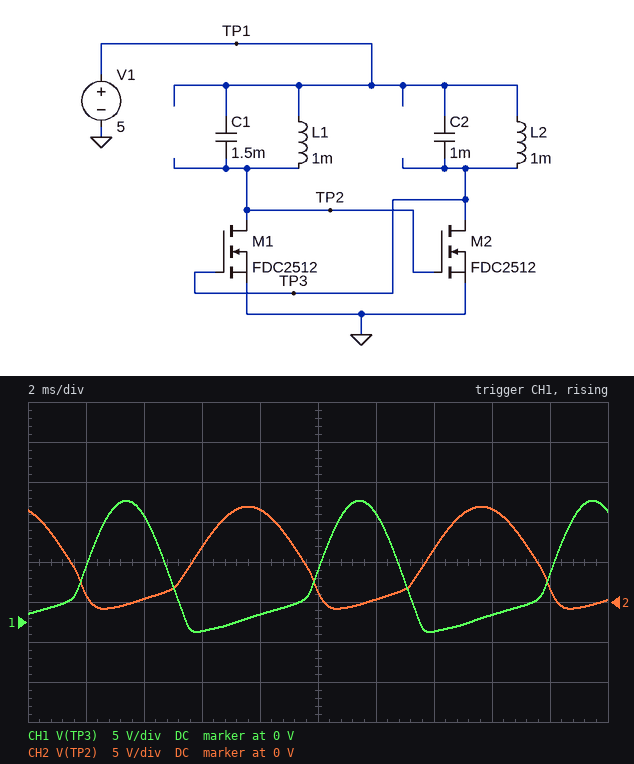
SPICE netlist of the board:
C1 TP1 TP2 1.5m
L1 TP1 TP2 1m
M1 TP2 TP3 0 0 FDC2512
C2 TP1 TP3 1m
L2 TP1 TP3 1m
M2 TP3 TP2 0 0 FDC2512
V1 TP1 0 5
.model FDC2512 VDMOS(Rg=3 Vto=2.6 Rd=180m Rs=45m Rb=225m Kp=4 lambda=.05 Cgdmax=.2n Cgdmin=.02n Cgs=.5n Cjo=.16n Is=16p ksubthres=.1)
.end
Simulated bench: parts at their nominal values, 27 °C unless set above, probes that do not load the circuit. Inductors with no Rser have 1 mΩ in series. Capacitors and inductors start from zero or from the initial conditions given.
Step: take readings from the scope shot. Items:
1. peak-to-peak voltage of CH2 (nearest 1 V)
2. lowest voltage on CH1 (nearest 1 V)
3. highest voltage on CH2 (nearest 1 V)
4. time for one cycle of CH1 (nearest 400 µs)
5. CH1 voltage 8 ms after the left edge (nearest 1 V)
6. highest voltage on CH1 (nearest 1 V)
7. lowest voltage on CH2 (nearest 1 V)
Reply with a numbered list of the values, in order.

1. 13 V
2. -1 V
3. 12 V
4. 8.0 ms
5. 1 V
6. 15 V
7. -1 V
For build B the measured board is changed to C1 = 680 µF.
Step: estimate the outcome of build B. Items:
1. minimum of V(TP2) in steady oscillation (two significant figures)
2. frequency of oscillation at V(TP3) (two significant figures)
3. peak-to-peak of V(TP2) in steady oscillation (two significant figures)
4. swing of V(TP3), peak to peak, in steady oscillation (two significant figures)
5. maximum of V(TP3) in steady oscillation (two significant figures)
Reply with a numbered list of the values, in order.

1. -1.2 V
2. 150 Hz
3. 17 V
4. 13 V
5. 12 V
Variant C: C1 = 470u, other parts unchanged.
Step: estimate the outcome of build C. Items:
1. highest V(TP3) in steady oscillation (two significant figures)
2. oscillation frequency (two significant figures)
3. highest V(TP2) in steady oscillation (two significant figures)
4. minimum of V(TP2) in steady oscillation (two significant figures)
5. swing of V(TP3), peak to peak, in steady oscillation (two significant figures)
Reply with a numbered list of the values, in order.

1. 11 V
2. 160 Hz
3. 18 V
4. -1.5 V
5. 12 V
